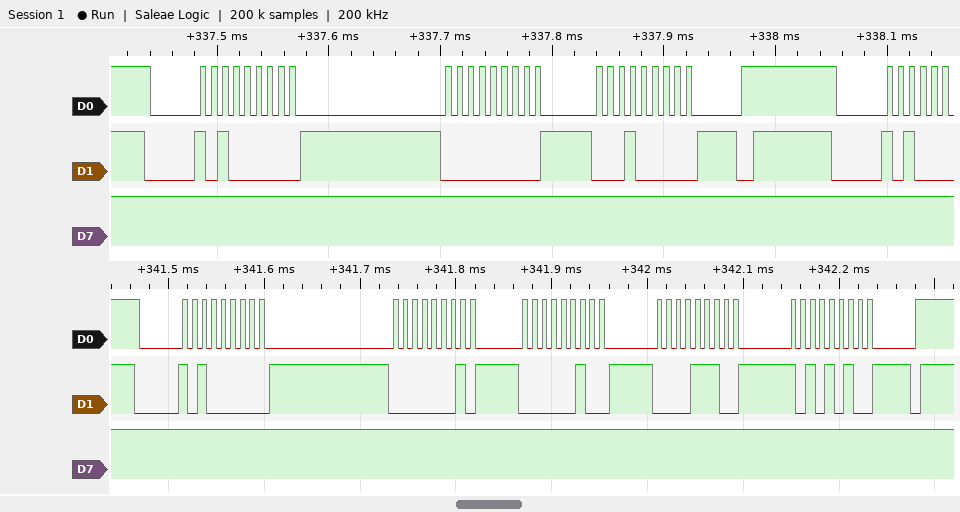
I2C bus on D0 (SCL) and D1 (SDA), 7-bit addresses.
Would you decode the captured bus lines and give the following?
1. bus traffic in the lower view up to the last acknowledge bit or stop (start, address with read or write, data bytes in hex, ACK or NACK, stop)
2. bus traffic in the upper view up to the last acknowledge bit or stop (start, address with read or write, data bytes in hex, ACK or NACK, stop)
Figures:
start, address 50 write ACK, 01 ACK, 02 ACK, 0E ACK, AA ACK, stop
start, address 50 write ACK, 00 ACK, 10 ACK, stop
